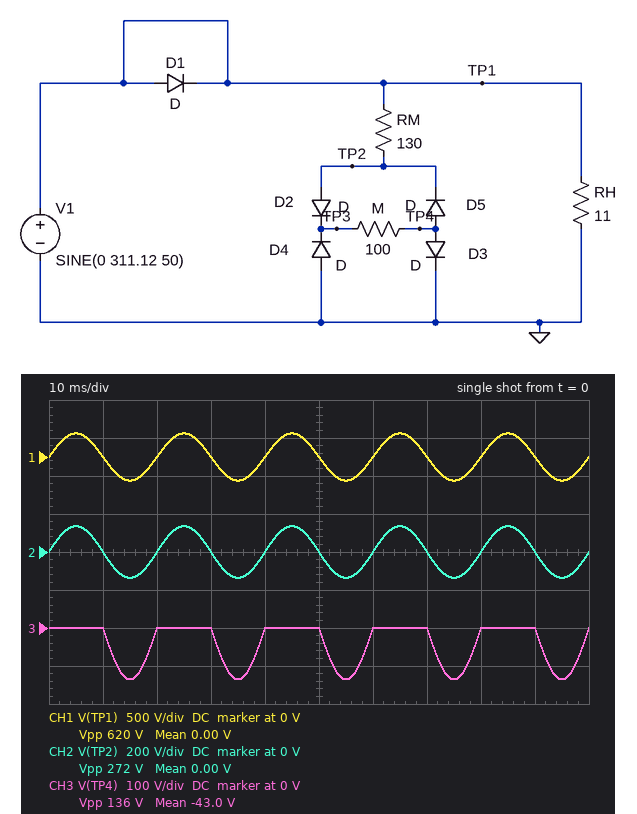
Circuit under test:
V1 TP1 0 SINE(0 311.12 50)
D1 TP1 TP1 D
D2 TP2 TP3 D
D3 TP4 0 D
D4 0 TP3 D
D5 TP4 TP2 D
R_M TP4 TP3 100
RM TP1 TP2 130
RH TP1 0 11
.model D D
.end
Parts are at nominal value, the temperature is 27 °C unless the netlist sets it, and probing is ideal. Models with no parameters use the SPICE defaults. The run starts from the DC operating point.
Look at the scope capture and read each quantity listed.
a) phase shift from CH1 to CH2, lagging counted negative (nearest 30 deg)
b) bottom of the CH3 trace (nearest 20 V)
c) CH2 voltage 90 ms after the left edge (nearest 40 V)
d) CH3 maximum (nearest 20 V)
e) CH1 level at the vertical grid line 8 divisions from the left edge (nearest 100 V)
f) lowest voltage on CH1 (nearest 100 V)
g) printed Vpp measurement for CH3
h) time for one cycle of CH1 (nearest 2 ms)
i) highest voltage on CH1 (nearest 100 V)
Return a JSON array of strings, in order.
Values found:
["0 deg", "-140 V", "0 V", "0 V", "0 V", "-300 V", "136 V", "20 ms", "300 V"]
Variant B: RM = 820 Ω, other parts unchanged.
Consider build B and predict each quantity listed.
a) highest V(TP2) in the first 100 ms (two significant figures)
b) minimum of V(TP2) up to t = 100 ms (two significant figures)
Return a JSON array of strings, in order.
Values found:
["35 V", "-35 V"]
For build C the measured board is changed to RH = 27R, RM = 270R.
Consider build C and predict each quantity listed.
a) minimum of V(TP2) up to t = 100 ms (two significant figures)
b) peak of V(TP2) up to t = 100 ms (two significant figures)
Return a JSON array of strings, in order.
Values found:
["-85 V", "85 V"]
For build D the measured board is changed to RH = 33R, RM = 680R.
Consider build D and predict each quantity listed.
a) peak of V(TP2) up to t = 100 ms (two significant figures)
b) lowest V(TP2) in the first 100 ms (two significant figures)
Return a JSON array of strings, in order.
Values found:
["41 V", "-41 V"]
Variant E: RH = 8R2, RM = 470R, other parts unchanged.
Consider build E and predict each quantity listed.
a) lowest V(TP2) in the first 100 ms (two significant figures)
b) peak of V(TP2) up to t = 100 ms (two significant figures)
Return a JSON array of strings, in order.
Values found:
["-56 V", "56 V"]
